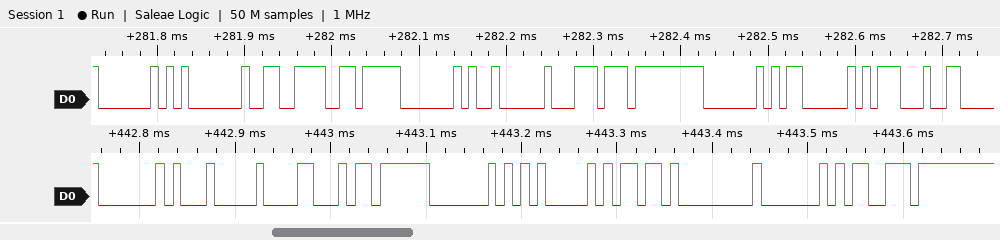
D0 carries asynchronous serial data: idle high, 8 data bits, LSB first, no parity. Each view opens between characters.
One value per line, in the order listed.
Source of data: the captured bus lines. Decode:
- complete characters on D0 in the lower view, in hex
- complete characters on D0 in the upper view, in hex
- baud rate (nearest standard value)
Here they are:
40, 04, 18, FB, 40, 05, 6D, 00, 40, 73
40, 01, E6, F6, 40, 02, DC, FF, 40, 03, 1D
115200 baud
